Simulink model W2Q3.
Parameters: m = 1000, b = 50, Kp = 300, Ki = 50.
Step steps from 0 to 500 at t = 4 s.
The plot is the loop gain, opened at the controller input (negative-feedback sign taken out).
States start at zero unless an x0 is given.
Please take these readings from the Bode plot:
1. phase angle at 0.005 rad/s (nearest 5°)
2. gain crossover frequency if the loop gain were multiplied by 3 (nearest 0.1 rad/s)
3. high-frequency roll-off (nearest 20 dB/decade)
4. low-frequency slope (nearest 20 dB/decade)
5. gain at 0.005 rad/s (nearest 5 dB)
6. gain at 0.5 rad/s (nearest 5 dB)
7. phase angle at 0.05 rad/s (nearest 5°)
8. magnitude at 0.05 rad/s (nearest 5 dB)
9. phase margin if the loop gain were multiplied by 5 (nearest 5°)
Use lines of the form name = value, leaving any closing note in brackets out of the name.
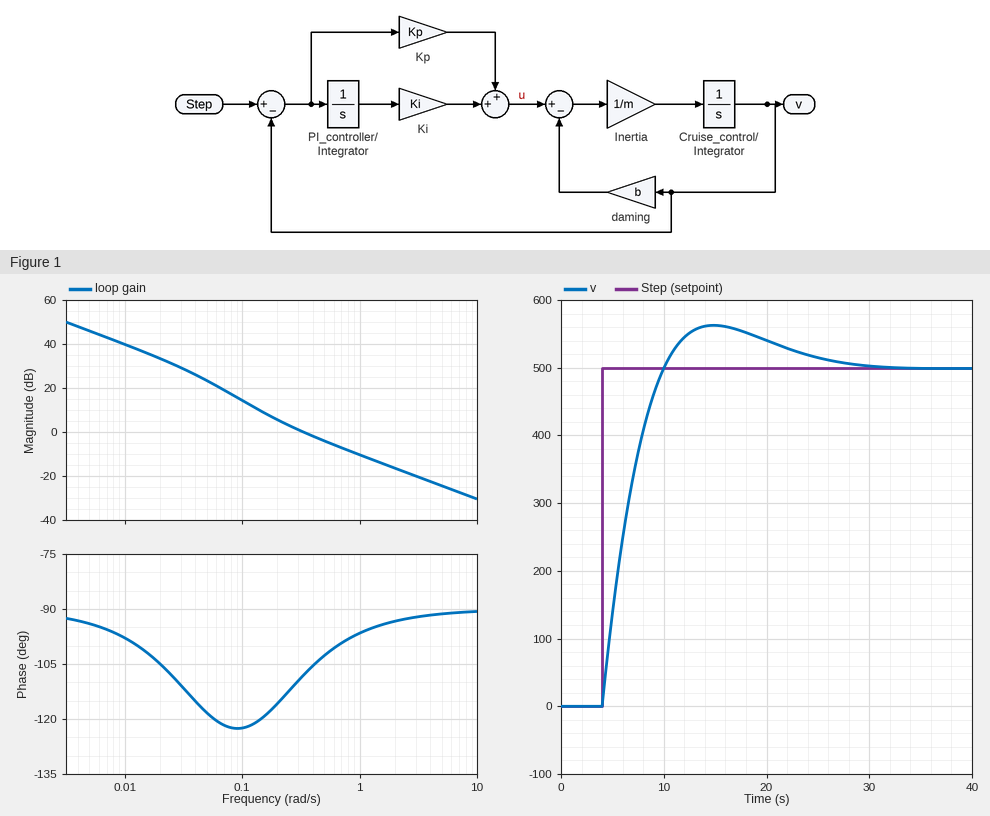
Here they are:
phase angle at 0.005 rad/s = -95°
gain crossover frequency if the loop gain were multiplied by 3 = 0.9 rad/s
high-frequency roll-off = -20 dB/decade
low-frequency slope = -20 dB/decade
gain at 0.005 rad/s = 45 dB
gain at 0.5 rad/s = -5 dB
phase angle at 0.05 rad/s = -120°
magnitude at 0.05 rad/s = 25 dB
phase margin if the loop gain were multiplied by 5 = 85°
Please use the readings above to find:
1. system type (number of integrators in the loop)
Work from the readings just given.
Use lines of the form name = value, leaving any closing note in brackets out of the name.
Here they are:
system type = 1
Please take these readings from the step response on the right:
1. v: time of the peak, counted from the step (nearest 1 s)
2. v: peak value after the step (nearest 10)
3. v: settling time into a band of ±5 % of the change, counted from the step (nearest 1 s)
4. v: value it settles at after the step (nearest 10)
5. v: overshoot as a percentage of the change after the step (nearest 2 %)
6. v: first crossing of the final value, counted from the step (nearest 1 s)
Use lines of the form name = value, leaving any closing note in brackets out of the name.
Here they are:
v: time of the peak, counted from the step = 11 s
v: peak value after the step = 560
v: settling time into a band of ±5 % of the change, counted from the step = 19 s
v: value it settles at after the step = 500
v: overshoot as a percentage of the change after the step = 12 %
v: first crossing of the final value, counted from the step = 6 s
